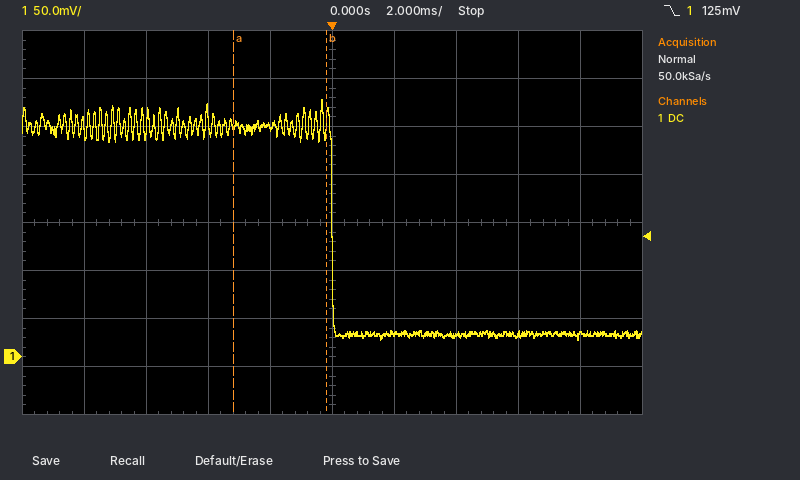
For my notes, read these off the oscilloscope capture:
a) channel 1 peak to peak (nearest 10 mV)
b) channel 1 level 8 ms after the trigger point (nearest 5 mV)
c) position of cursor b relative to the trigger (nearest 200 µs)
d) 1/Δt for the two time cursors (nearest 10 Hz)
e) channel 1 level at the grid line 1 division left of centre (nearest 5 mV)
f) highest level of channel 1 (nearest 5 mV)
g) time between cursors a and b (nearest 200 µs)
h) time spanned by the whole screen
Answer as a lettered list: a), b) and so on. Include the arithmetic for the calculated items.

a) 250 mV
b) 20 mV
c) -200 µs
d) 1 / 3.0 ms ≈ 330 Hz
e) 240 mV
f) 270 mV
g) 3.0 ms
h) 20 ms
